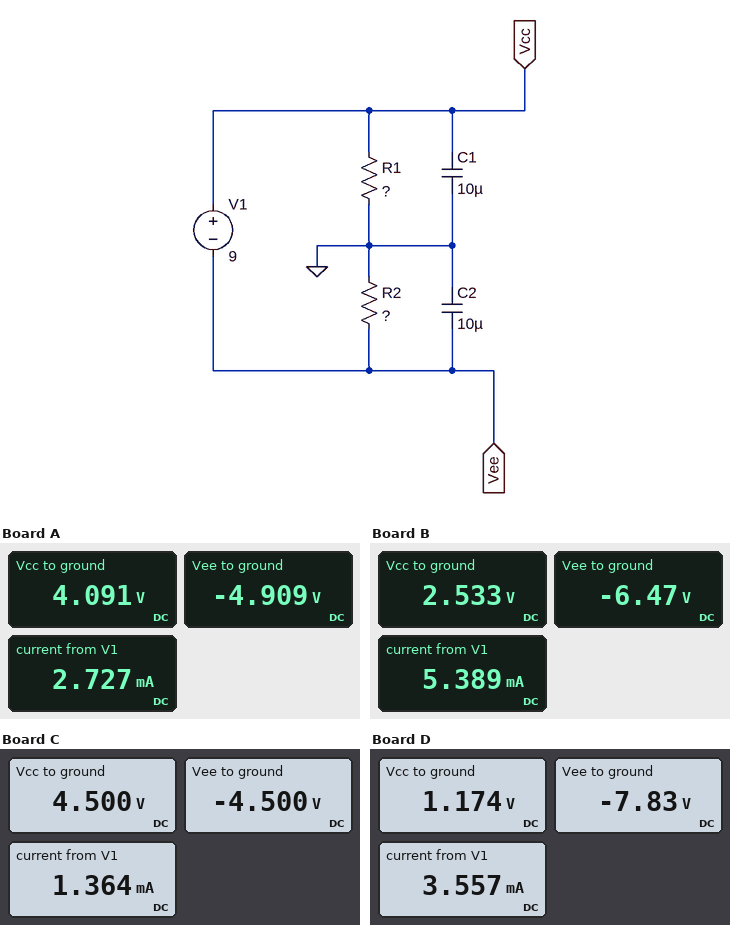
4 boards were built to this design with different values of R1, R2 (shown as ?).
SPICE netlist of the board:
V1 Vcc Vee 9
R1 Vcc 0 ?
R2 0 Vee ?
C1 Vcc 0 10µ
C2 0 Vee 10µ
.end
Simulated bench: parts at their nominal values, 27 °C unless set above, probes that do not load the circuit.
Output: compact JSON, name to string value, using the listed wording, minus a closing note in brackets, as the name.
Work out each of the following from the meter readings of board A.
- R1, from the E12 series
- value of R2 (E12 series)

{"R1, from the E12 series": "1.5 kΩ", "value of R2": "1.8 kΩ"}
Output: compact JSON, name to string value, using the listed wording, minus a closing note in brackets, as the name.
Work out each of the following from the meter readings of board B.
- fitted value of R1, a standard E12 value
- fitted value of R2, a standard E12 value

{"fitted value of R1, a standard E12 value": "470 Ω", "fitted value of R2, a standard E12 value": "1.2 kΩ"}
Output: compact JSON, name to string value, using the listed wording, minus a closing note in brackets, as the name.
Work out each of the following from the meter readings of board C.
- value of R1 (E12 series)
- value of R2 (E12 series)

{"value of R1": "3.3 kΩ", "value of R2": "3.3 kΩ"}
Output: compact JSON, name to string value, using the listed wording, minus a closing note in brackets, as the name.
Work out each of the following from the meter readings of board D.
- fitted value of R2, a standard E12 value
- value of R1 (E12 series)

{"fitted value of R2, a standard E12 value": "2.2 kΩ", "value of R1": "330 Ω"}
